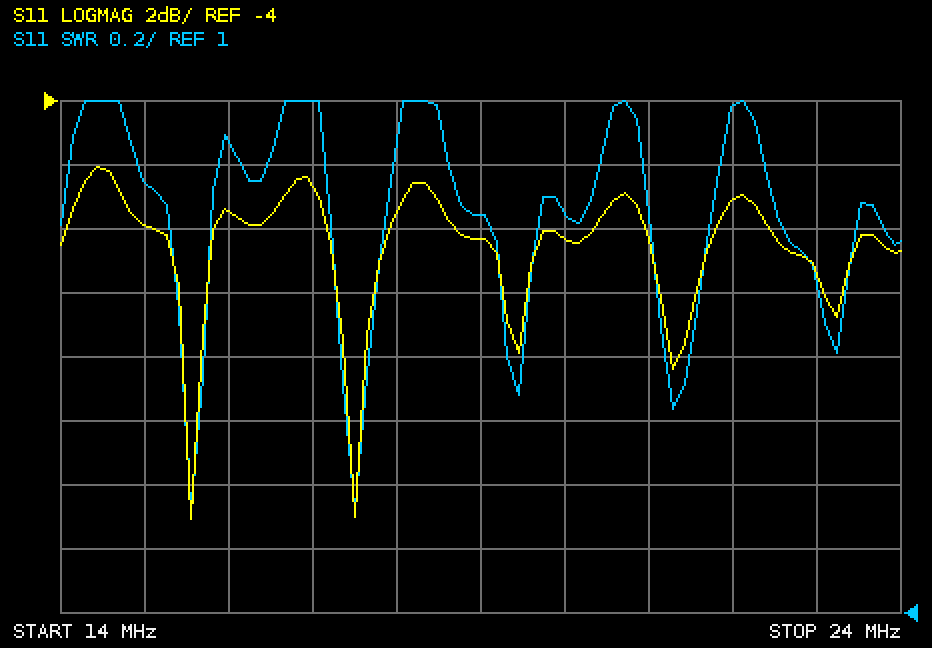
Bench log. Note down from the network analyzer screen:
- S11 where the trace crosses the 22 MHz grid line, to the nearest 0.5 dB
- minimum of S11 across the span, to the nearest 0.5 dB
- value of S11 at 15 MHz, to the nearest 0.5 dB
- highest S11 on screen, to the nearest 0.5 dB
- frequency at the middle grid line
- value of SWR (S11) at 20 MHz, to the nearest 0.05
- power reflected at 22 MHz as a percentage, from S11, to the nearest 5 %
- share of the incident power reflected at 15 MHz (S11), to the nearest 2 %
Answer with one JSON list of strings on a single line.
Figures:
["-7.0 dB", "-17.0 dB", "-8.0 dB", "-6.0 dB", "19 MHz", "2.25", "20 %", "16 %"]
